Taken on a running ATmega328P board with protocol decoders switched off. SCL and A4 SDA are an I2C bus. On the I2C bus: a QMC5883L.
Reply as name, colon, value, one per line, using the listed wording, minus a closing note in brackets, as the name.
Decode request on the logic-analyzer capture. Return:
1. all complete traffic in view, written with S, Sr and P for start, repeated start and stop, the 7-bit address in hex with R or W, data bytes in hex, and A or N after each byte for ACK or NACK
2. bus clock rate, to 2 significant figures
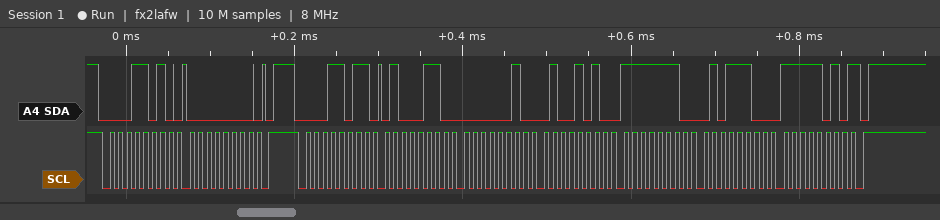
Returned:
all complete traffic in view, written with S, Sr and P for start, repeated start and stop, the 7-bit address in hex with R or W, data bytes in hex, and A or N after each byte for ACK or NACK: S 0DW A 00 A P S 0DR A 46 A 02 A 4A A FE A 5C A FA N P
bus clock rate, to 2 significant figures: 100 kHz
